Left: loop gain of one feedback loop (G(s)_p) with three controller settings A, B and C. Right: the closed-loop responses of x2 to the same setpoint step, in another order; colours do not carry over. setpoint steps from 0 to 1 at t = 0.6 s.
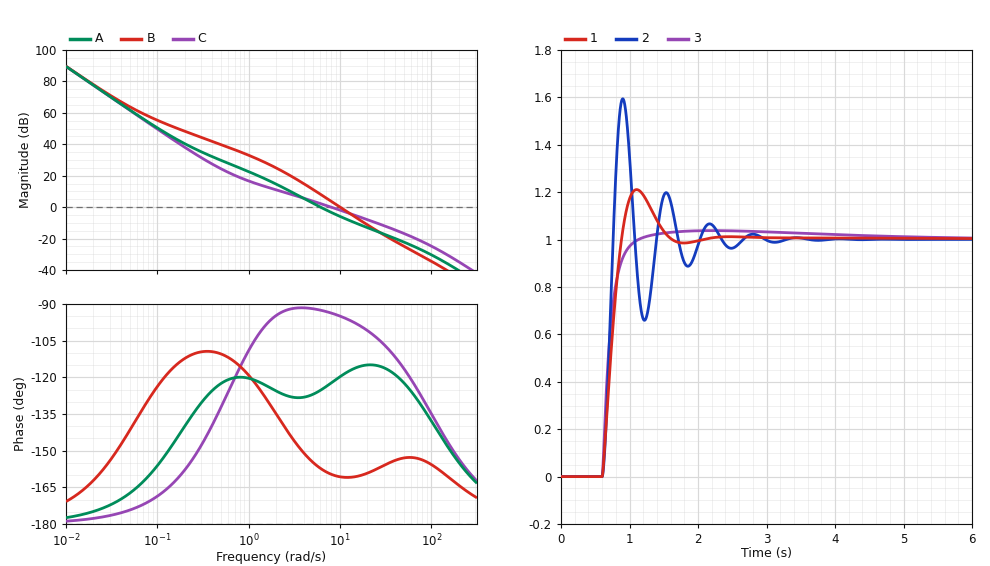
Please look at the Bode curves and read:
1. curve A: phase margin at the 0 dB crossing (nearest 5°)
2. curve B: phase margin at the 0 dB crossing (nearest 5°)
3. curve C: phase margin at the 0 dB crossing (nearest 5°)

55°
20°
85°
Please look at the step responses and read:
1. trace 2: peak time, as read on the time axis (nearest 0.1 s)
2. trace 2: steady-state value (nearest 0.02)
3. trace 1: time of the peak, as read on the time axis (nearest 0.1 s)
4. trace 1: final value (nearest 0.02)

0.9 s
1.00
1.1 s
1.00
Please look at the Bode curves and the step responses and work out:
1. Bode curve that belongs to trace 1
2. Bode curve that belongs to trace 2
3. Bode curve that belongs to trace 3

A
B
C
